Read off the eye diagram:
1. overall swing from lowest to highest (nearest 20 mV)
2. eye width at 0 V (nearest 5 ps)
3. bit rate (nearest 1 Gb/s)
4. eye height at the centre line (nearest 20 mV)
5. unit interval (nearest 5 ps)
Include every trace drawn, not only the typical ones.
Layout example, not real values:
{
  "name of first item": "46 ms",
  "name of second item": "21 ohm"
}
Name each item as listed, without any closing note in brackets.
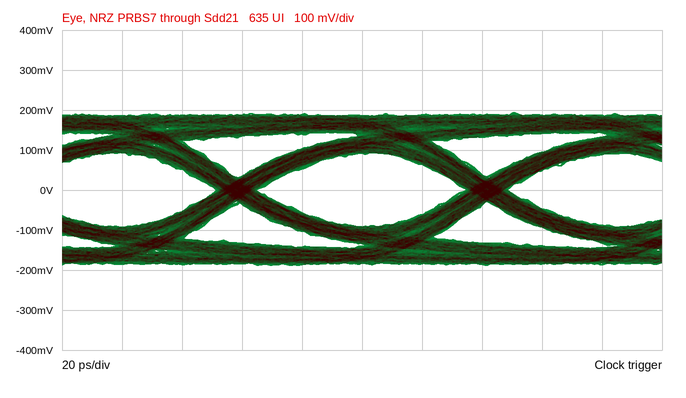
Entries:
{
  "overall swing from lowest to highest": "380 mV",
  "eye width at 0 V": "70 ps",
  "bit rate": "12 Gb/s",
  "eye height at the centre line": "180 mV",
  "unit interval": "85 ps"
}
